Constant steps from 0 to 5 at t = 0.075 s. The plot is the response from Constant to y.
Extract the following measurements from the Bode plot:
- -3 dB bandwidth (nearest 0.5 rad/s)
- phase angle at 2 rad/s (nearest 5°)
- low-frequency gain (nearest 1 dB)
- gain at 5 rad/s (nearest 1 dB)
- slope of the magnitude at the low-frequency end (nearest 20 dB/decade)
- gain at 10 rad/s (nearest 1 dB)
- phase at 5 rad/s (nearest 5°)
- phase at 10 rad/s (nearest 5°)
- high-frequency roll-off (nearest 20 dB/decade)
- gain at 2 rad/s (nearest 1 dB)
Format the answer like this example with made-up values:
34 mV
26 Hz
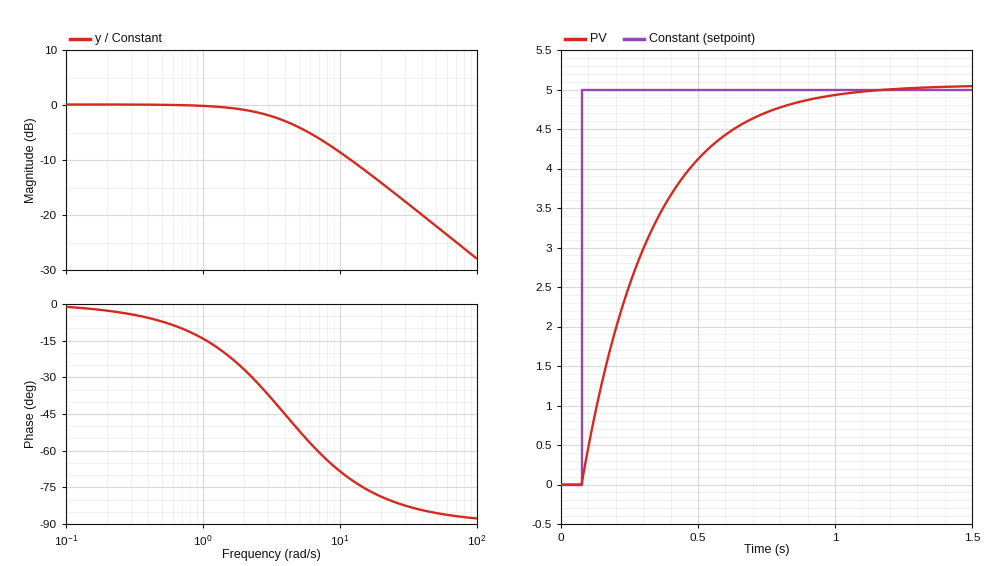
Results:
4.0 rad/s
-25°
0 dB
-4 dB
0 dB/decade
-9 dB
-50°
-70°
-20 dB/decade
-1 dB
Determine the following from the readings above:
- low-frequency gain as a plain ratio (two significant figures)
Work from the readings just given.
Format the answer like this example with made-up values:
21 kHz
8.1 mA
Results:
1.0
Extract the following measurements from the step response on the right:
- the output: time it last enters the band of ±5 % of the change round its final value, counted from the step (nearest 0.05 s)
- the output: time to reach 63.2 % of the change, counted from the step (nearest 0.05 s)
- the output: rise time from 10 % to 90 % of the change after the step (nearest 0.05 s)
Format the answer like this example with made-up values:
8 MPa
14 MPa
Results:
0.75 s
0.25 s
0.55 s
